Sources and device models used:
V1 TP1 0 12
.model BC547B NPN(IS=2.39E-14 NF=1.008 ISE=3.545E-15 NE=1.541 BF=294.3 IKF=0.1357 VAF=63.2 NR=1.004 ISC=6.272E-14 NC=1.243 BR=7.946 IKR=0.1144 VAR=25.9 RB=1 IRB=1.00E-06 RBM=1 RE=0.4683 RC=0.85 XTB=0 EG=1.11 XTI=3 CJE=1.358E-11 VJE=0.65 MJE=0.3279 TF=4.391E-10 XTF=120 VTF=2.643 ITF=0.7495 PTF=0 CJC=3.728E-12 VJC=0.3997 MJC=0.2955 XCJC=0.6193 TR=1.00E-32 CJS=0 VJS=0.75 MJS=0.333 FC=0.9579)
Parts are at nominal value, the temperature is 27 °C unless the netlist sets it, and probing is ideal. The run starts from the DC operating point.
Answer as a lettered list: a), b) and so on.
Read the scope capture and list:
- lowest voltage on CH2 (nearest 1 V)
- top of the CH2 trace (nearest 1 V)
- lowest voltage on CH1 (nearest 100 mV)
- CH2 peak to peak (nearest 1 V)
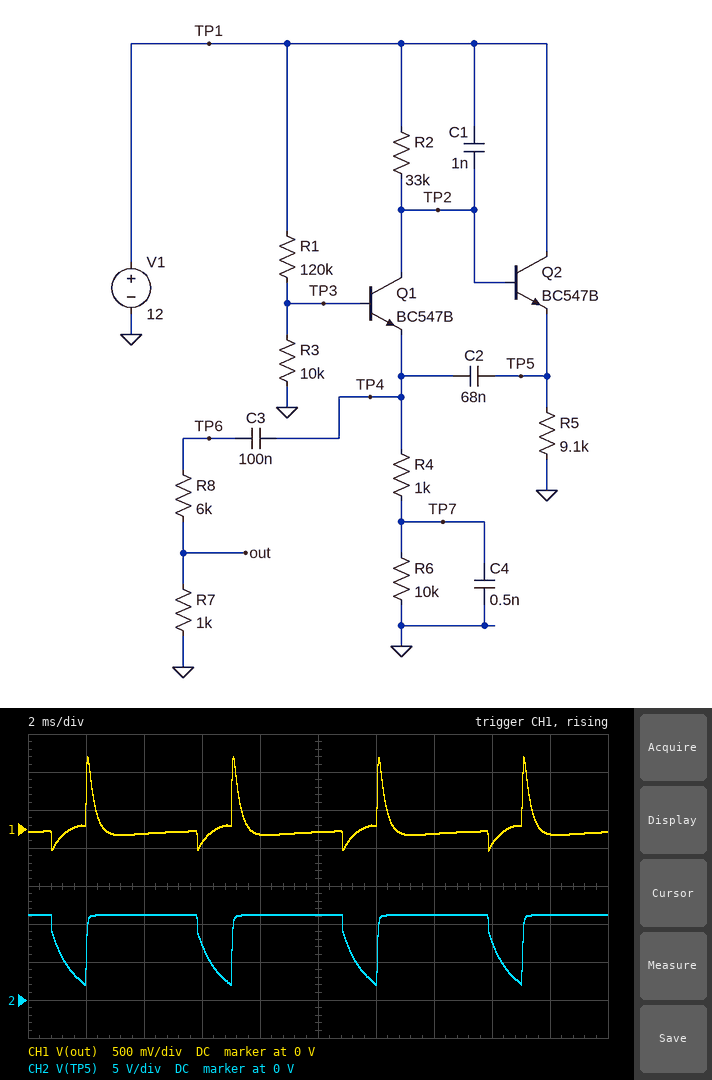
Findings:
a) 2 V
b) 11 V
c) -300 mV
d) 9 V
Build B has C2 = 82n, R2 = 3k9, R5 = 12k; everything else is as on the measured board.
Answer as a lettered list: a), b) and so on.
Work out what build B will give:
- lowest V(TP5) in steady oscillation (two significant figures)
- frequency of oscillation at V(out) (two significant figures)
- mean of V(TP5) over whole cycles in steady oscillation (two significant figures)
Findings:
a) 8.7 V
b) 380 Hz
c) 11 V
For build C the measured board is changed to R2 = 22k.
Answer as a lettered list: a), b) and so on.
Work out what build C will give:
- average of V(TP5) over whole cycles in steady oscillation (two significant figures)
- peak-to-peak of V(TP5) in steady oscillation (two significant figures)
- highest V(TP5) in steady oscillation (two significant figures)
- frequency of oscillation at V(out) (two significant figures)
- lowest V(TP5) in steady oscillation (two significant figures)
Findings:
a) 10 V
b) 8.2 V
c) 11 V
d) 220 Hz
e) 3.0 V
